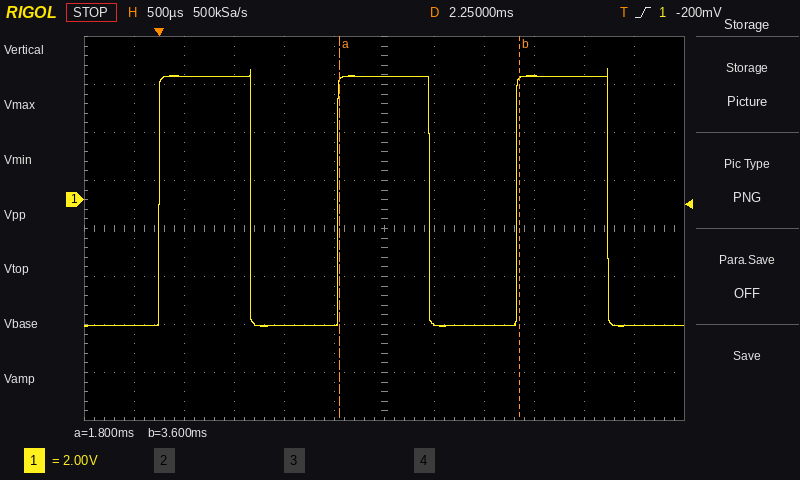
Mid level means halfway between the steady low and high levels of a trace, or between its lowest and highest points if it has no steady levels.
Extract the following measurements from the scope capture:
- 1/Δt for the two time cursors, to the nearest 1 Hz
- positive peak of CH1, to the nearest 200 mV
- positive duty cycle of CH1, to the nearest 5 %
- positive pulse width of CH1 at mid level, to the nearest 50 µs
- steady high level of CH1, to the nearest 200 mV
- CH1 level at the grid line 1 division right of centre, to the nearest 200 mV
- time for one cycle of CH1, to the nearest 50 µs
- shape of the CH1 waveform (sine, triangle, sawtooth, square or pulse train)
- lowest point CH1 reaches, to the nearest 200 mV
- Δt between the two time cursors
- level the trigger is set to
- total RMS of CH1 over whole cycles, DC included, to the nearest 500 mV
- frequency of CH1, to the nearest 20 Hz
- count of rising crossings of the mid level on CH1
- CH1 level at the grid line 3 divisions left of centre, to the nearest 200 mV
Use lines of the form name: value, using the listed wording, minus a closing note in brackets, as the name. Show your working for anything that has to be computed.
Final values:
1/Δt for the two time cursors, to the nearest 1 Hz: 1 / 1.80 ms ≈ 556 Hz
positive peak of CH1, to the nearest 200 mV: 5.4 V
positive duty cycle of CH1, to the nearest 5 %: 900 µs / 1.80 ms ≈ 50 %
positive pulse width of CH1 at mid level, to the nearest 50 µs: 900 µs
steady high level of CH1, to the nearest 200 mV: 5.2 V
CH1 level at the grid line 1 division right of centre, to the nearest 200 mV: -5.2 V
time for one cycle of CH1, to the nearest 50 µs: 1.80 ms
shape of the CH1 waveform: square
lowest point CH1 reaches, to the nearest 200 mV: -5.2 V
Δt between the two time cursors: 3.6 ms − (1.8 ms) = 1.80 ms
level the trigger is set to: -200 mV
total RMS of CH1 over whole cycles, DC included, to the nearest 500 mV: √(0.5 × (5.2 V)² + 0.5 × (-5.2 V)²) ≈ 5.20 V, so 5.0 V to the nearest 500 mV
frequency of CH1, to the nearest 20 Hz: 1 / 1.80 ms ≈ 556 Hz, so 560 Hz to the nearest 20 Hz
count of rising crossings of the mid level on CH1: 3
CH1 level at the grid line 3 divisions left of centre, to the nearest 200 mV: 5.2 V
